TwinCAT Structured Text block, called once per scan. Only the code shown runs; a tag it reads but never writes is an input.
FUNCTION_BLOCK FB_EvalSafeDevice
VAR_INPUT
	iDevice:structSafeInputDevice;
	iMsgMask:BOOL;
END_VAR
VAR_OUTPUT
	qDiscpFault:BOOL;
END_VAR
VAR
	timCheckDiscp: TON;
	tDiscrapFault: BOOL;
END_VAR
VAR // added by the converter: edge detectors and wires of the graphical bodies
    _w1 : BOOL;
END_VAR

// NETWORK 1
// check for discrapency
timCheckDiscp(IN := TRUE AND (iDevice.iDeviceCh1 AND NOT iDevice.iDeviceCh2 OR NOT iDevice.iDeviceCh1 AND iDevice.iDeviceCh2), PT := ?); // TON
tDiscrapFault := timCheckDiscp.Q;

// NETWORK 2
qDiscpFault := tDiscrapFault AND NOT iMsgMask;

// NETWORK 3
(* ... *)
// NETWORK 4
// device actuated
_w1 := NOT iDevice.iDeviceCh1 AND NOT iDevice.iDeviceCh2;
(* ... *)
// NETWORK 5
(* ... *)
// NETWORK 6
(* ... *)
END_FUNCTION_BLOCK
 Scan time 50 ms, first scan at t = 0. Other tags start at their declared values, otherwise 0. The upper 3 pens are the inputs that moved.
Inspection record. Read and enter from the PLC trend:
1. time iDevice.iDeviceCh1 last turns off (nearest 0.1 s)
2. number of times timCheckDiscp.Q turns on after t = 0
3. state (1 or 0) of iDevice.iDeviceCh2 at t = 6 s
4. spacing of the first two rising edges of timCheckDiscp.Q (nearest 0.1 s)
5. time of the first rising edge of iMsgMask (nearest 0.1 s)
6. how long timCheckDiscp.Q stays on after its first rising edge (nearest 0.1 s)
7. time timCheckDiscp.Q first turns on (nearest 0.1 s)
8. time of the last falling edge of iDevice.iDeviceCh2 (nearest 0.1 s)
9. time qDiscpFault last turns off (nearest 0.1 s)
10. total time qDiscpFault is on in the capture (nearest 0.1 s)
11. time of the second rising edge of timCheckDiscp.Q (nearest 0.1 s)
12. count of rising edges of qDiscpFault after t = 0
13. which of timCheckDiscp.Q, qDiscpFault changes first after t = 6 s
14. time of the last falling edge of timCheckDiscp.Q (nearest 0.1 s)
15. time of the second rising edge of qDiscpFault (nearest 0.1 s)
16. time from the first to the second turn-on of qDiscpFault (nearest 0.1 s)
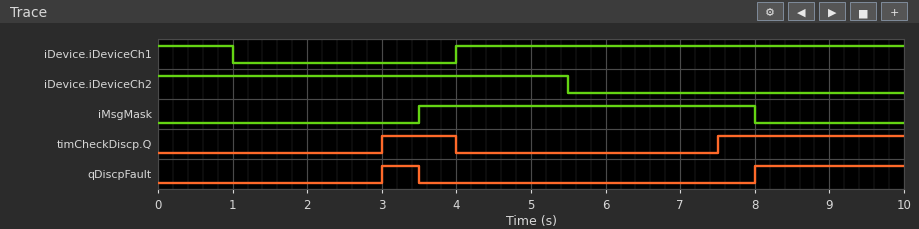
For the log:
1.0 s
2
0
4.5 s
3.5 s
1.0 s
3.0 s
5.5 s
3.5 s
2.5 s
7.5 s
2
timCheckDiscp.Q
4.0 s
8.0 s
5.0 s
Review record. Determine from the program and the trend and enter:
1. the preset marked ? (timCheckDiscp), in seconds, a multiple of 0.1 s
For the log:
2.0 s
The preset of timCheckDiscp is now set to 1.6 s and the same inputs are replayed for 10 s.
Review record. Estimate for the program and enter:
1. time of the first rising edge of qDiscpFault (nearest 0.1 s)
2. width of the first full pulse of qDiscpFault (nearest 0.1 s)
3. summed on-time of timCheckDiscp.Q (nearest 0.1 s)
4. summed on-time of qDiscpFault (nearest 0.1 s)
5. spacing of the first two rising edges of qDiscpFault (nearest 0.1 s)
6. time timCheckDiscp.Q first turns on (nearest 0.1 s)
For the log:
2.6 s
0.9 s
4.3 s
2.9 s
5.4 s
2.6 s
